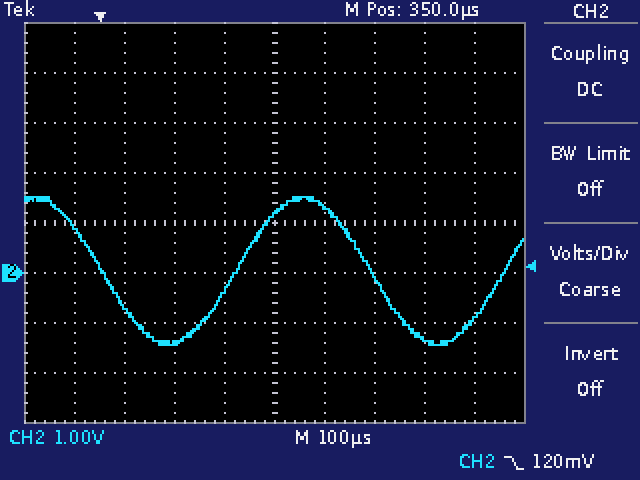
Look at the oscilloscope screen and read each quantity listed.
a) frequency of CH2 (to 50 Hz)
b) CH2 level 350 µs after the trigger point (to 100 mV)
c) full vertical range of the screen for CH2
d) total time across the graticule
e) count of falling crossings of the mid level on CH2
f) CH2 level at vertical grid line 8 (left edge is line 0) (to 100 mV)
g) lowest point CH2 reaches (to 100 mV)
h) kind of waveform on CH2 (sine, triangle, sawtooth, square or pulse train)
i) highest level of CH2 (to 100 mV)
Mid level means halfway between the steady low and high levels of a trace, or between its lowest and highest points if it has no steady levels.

1.85 kHz
1.2 V
8 V
1 ms
2
-1.3 V
-1.4 V
sine
1.5 V
